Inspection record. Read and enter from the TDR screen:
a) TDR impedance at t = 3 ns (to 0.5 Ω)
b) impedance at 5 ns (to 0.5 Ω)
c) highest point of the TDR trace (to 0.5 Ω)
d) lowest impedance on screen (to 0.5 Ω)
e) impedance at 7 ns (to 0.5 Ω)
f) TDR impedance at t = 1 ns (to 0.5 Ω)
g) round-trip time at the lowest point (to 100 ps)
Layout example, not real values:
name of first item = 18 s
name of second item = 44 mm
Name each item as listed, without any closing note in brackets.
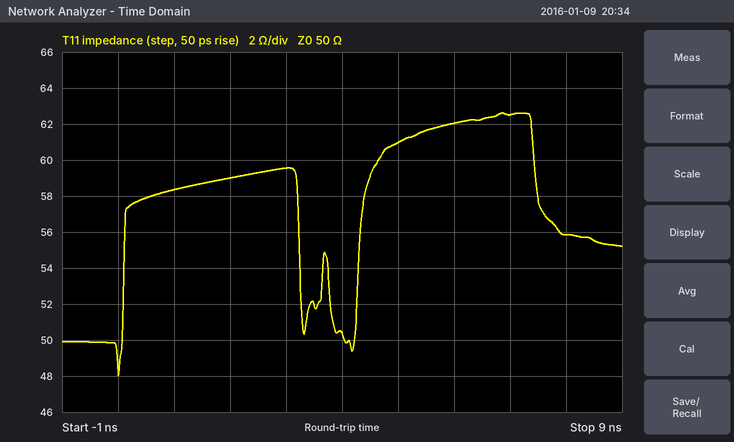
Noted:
TDR impedance at t = 3 ns = 59.5 Ω
impedance at 5 ns = 61.0 Ω
highest point of the TDR trace = 62.5 Ω
lowest impedance on screen = 48.0 Ω
impedance at 7 ns = 62.5 Ω
TDR impedance at t = 1 ns = 58.5 Ω
round-trip time at the lowest point = 0.0 ns
